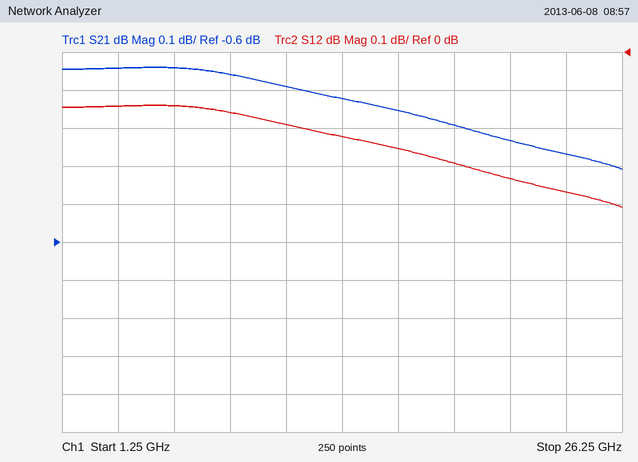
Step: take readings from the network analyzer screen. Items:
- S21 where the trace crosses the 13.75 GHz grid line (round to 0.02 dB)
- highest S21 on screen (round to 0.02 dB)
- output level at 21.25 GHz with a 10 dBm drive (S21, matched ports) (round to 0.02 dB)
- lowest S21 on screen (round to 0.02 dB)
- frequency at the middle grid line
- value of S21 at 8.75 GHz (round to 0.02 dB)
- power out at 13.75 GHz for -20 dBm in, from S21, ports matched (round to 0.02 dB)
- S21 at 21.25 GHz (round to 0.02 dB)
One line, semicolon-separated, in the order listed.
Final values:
-0.22 dB; -0.14 dB; 9.66 dBm; -0.40 dB; 13.75 GHz; -0.16 dB; -20.22 dBm; -0.34 dB
